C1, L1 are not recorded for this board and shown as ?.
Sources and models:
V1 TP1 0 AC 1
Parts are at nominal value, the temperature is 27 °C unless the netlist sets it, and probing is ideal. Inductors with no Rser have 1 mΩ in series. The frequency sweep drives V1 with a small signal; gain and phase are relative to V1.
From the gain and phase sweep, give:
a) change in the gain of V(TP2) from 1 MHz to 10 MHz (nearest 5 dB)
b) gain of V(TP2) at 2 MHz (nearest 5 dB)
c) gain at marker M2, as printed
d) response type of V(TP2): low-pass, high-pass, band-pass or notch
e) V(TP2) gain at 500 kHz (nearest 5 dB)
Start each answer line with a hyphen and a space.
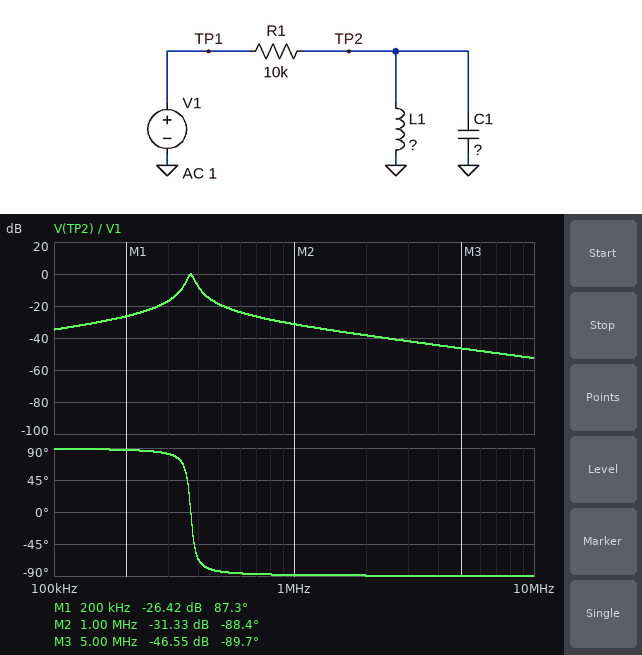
- -20 dB
- -40 dB
- -31.33 dB
- band-pass
- -20 dB
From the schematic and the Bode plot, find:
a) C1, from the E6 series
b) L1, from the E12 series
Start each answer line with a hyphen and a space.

- 680 pF
- 270 µH
